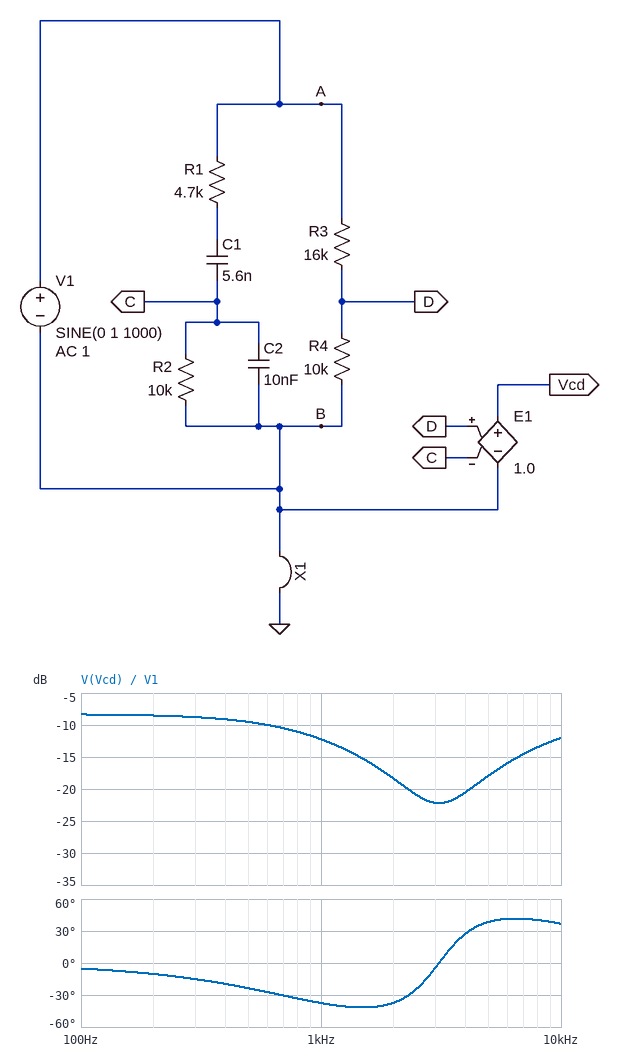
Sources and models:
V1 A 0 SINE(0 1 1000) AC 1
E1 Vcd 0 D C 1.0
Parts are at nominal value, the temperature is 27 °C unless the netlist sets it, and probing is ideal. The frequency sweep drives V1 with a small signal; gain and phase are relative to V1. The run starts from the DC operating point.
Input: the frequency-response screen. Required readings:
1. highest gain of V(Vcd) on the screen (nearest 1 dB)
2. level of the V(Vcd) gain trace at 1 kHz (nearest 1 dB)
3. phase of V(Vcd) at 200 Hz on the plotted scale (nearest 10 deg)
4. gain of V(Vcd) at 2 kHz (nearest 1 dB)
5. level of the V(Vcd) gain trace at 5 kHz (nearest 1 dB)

-8 dB
-12 dB
-10 deg
-18 dB
-18 dB
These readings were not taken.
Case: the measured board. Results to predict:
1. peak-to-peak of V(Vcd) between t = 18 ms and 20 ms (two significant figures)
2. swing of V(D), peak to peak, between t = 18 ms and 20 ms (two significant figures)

490 mV
770 mV
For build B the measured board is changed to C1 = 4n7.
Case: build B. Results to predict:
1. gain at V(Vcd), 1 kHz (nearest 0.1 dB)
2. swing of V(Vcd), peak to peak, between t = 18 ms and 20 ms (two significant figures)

-11.6 dB
530 mV
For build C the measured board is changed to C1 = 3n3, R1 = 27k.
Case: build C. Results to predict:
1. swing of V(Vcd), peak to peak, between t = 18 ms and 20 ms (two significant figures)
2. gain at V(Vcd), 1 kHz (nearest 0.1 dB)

540 mV
-11.4 dB
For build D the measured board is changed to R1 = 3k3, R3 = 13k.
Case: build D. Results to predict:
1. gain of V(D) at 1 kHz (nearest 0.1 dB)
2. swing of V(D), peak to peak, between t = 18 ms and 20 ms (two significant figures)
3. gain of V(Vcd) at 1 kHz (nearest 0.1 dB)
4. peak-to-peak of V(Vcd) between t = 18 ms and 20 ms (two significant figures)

-7.2 dB
870 mV
-10.6 dB
590 mV
